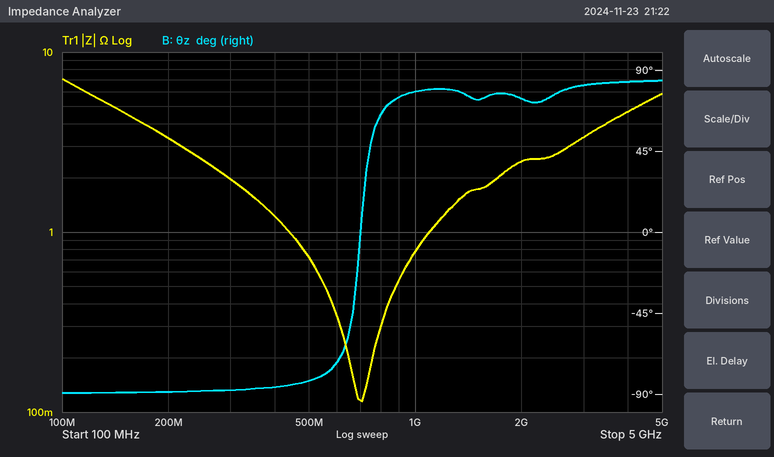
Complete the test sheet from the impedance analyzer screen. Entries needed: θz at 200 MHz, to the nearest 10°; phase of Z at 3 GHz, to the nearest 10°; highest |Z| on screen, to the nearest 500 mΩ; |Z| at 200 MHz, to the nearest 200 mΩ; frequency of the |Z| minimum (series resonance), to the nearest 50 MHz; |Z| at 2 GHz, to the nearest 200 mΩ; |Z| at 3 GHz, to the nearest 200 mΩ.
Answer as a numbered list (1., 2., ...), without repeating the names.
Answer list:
1. -90°
2. 80°
3. 7.0 Ω
4. 3.4 Ω
5. 700 MHz
6. 2.4 Ω
7. 3.4 Ω
